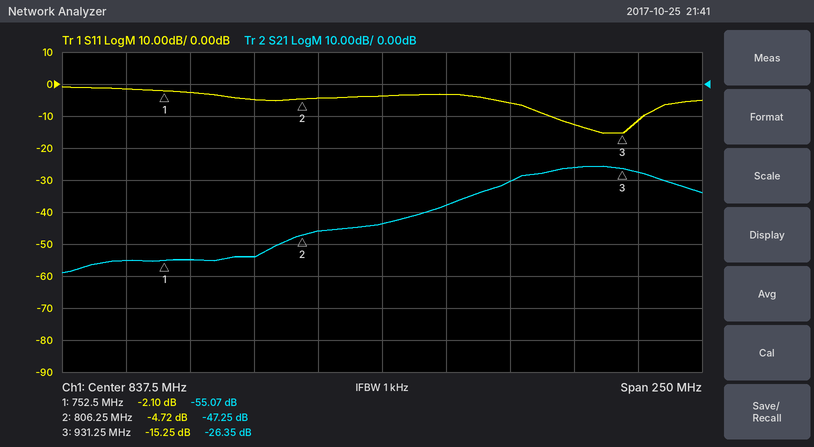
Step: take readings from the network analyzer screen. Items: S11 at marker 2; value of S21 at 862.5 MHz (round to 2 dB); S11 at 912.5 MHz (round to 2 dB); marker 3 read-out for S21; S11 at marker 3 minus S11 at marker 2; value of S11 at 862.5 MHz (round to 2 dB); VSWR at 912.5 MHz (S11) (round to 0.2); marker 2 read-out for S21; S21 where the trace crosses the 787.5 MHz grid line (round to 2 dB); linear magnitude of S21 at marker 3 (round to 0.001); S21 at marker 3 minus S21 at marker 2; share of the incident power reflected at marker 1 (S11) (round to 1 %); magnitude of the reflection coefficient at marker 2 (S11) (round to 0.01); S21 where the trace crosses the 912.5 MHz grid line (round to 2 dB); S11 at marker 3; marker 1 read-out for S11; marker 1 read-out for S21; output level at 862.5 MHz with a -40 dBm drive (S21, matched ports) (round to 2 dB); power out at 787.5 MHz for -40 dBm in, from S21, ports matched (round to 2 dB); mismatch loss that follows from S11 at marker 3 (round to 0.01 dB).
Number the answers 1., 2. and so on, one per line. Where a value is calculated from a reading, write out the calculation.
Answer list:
1. -4.72 dB
2. -38 dB
3. -12 dB
4. -26.35 dB
5. -15.25 − (-4.72) = -10.53 dB
6. -4 dB
7. |Γ| = 10^(-12/20) = 0.2512; VSWR = (1 + 0.2512)/(1 − 0.2512) ≈ 1.67, so 1.6 to the nearest 0.2
8. -47.25 dB
9. -54 dB
10. 10^(-26.35/20) ≈ 0.048
11. -26.35 − (-47.25) = 20.90 dB
12. 10^(-2.1/10) ≈ 62 %
13. 10^(-4.72/20) ≈ 0.58
14. -26 dB
15. -15.25 dB
16. -2.10 dB
17. -55.07 dB
18. -40 dBm + (-38 dB) = -78 dBm
19. -40 dBm + (-54 dB) = -94 dBm
20. −10 log10(1 − 10^(-15.25/10)) ≈ 0.13 dB
